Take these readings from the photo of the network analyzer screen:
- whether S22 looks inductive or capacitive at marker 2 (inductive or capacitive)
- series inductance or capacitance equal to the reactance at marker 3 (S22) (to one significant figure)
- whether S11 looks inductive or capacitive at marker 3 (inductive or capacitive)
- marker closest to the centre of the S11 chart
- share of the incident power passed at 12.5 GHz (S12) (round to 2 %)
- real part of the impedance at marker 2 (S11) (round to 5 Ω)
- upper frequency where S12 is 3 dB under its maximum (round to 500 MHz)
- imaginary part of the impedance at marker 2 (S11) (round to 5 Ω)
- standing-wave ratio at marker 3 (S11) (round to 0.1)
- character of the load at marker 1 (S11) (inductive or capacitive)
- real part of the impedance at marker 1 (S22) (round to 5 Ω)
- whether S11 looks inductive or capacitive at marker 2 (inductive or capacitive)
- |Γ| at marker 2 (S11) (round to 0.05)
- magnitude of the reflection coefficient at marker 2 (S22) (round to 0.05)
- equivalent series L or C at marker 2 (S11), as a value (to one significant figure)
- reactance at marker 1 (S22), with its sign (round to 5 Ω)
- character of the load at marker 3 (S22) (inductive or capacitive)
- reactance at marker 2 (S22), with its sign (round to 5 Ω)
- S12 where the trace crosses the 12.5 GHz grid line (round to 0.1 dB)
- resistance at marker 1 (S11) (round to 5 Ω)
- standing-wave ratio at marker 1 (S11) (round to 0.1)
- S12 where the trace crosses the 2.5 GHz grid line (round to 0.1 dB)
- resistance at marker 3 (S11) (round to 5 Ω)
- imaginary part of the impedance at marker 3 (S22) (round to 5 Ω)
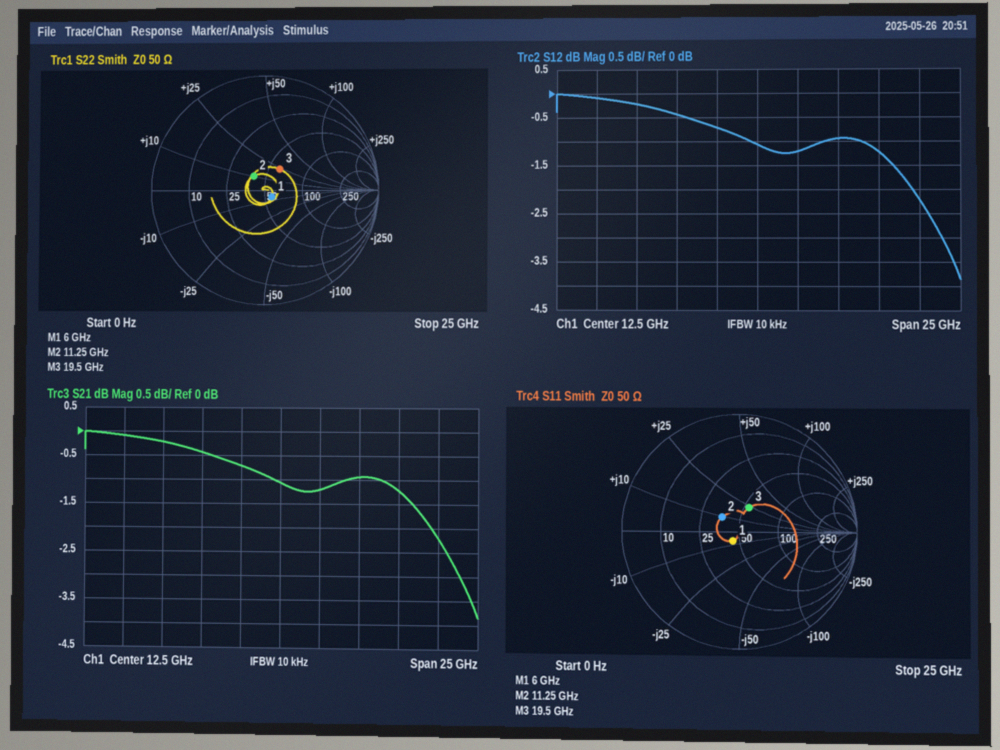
inductive
200 pH
inductive
marker 1
78 %
35 Ω
24.0 GHz
+10 Ω
1.6
capacitive
55 Ω
inductive
0.20
0.15
100 pH
-5 Ω
inductive
+10 Ω
-1.1 dB
45 Ω
1.2
-0.1 dB
55 Ω
+25 Ω
